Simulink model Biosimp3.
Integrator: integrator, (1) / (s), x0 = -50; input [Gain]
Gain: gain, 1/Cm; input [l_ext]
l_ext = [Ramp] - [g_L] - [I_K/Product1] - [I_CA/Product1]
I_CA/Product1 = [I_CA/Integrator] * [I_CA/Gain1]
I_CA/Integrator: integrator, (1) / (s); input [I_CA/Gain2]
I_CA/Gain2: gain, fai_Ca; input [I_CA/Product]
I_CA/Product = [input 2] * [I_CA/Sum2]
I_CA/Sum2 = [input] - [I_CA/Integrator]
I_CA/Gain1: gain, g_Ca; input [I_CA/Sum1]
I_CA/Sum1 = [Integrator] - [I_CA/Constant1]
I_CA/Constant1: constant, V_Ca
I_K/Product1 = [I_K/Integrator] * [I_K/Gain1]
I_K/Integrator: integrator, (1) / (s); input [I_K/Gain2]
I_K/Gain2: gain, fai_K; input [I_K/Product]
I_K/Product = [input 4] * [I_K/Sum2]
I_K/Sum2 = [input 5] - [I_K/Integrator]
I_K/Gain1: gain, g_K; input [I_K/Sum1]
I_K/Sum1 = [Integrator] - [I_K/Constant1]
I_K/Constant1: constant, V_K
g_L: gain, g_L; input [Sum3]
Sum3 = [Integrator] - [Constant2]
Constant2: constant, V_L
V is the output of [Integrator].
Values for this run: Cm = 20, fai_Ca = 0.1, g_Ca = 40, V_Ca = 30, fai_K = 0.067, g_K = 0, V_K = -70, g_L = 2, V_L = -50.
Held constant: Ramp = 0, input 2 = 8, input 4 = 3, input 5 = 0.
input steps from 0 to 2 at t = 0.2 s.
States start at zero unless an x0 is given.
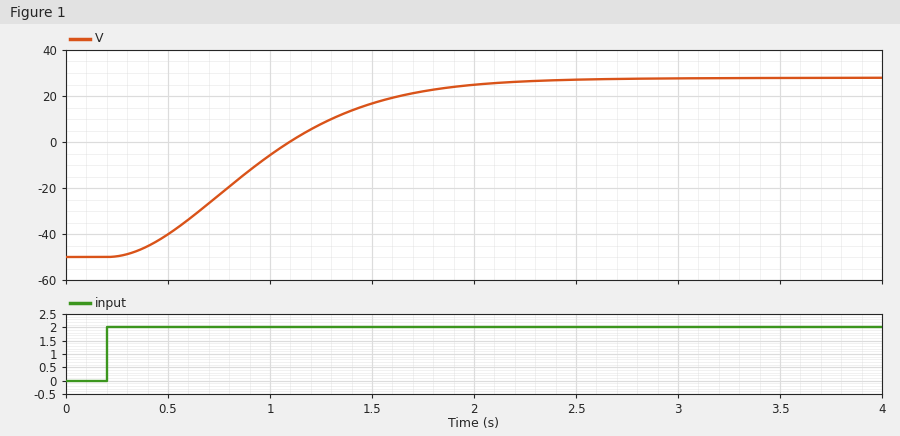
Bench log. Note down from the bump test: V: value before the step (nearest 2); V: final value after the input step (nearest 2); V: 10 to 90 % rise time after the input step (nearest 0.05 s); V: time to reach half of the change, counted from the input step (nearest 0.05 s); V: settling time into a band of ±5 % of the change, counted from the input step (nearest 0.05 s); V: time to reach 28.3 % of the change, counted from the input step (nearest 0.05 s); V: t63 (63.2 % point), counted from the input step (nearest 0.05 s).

-50
28
1.20 s
0.70 s
1.70 s
0.50 s
0.90 s
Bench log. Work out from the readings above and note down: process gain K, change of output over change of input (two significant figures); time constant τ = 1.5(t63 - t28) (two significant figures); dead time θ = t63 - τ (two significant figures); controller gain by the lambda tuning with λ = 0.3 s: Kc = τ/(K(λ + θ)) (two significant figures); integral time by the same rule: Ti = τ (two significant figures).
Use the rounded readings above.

39
0.60 s
0.30 s
0.026
0.60 s
